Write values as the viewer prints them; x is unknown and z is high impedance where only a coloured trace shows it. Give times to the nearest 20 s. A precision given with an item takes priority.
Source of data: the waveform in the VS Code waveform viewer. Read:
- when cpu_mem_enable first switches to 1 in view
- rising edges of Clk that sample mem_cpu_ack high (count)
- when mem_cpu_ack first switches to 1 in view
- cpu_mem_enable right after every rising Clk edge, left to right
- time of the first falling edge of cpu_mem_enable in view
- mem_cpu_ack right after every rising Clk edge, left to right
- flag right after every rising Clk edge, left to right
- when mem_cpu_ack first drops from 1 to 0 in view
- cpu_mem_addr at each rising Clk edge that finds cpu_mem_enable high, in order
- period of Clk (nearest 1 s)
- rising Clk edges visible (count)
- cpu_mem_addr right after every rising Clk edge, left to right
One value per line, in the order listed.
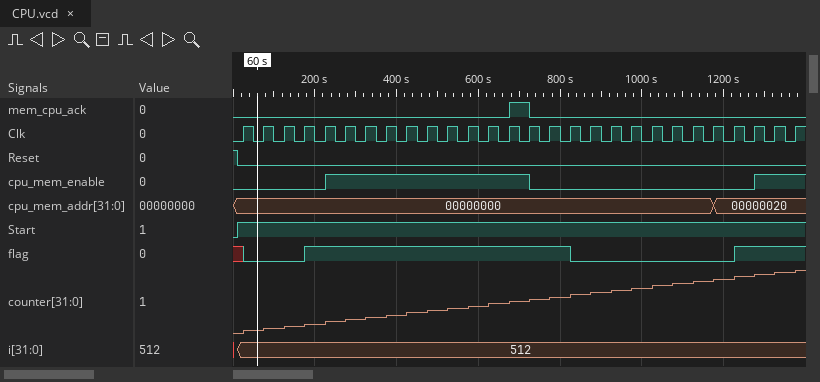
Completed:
220 s
1
680 s
0 0 0 0 1 1 1 1 1 1 1 1 1 1 0 0 0 0 0 0 0 0 0 0 0 1 1 1
720 s
0 0 0 0 0 0 0 0 0 0 0 0 0 1 0 0 0 0 0 0 0 0 0 0 0 0 0 0
0 0 0 1 1 1 1 1 1 1 1 1 1 1 1 1 0 0 0 0 0 0 0 0 1 1 1 1
720 s
00000000, 00000000, 00000000, 00000000, 00000000, 00000000, 00000000, 00000000, 00000000, 00000000, 00000020, 00000020
50 s
28
00000000, 00000000, 00000000, 00000000, 00000000, 00000000, 00000000, 00000000, 00000000, 00000000, 00000000, 00000000, 00000000, 00000000, 00000000, 00000000, 00000000, 00000000, 00000000, 00000000, 00000000, 00000000, 00000000, 00000020, 00000020, 00000020, 00000020, 00000020
